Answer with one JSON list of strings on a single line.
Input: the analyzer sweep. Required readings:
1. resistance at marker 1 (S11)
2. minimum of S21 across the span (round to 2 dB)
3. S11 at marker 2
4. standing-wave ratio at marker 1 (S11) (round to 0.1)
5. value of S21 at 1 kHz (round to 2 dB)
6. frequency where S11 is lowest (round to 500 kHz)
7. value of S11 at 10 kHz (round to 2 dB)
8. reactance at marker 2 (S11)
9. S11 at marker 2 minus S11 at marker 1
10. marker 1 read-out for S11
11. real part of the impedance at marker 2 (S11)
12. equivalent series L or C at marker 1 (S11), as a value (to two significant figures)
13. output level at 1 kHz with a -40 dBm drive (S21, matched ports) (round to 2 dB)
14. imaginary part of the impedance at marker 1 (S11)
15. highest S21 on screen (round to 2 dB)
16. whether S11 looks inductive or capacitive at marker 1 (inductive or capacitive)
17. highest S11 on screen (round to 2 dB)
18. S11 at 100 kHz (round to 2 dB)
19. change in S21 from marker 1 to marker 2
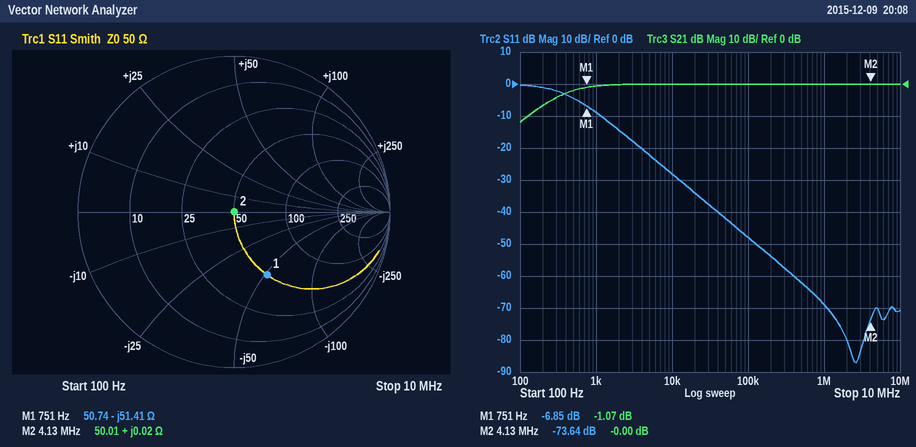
["50.74 Ω", "-12 dB", "-73.64 dB", "2.7", "0 dB", "2.5 MHz", "-28 dB", "+0.02 Ω", "-66.79 dB", "-6.85 dB", "50.01 Ω", "4.1 µF", "-40 dBm", "-51.41 Ω", "0 dB", "capacitive", "0 dB", "-48 dB", "1.07 dB"]
